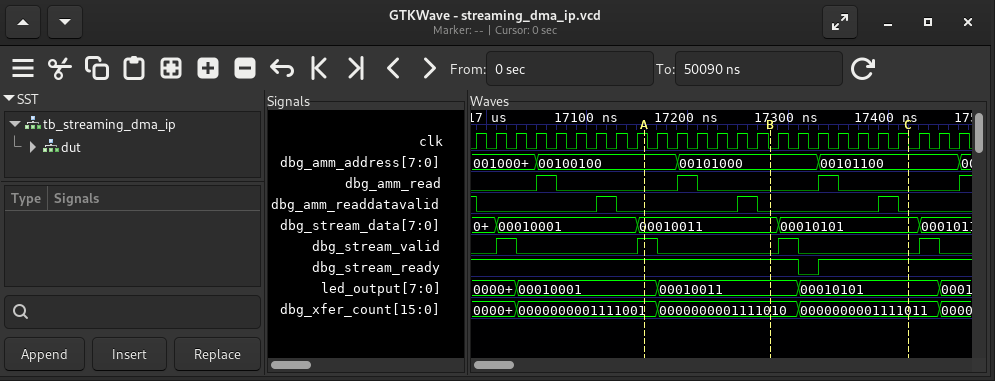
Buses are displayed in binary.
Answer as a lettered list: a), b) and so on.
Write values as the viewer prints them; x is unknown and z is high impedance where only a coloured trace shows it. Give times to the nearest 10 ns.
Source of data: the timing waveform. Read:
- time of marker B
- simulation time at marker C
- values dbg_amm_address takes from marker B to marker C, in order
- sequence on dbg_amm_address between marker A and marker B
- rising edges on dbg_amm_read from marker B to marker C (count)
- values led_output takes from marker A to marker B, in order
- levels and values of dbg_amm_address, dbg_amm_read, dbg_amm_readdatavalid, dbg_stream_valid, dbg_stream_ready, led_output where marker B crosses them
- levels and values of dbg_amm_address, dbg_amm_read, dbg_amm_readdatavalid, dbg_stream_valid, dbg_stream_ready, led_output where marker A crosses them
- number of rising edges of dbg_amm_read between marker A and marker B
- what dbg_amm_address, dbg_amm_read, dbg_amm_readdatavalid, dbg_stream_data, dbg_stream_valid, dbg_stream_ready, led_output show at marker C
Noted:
a) 17280 ns
b) 17420 ns
c) 00101000, 00101100
d) 00100100, 00101000
e) 1
f) 00010001, 00010011
g) dbg_amm_address=00101000, dbg_amm_read=0, dbg_amm_readdatavalid=0, dbg_stream_valid=0, dbg_stream_ready=1, led_output=00010011
h) dbg_amm_address=00100100, dbg_amm_read=0, dbg_amm_readdatavalid=0, dbg_stream_valid=1, dbg_stream_ready=1, led_output=00010001
i) 1
j) dbg_amm_address=00101100, dbg_amm_read=0, dbg_amm_readdatavalid=0, dbg_stream_data=00010101, dbg_stream_valid=0, dbg_stream_ready=1, led_output=00010101
